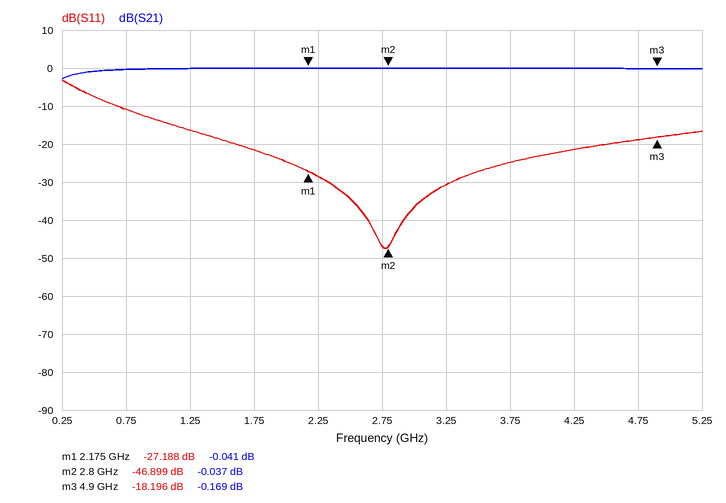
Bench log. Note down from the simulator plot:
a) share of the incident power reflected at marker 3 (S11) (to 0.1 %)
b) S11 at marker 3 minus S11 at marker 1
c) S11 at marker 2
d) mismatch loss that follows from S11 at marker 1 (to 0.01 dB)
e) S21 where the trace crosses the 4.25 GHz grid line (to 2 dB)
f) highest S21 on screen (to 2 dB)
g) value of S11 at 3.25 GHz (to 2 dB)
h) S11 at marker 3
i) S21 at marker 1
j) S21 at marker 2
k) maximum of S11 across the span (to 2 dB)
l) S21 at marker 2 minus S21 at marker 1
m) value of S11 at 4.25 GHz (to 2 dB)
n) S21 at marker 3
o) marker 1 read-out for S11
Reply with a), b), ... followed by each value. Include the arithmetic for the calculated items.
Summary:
a) 10^(-18.196/10) ≈ 1.5 %
b) -18.196 − (-27.188) = 8.992 dB
c) -46.899 dB
d) −10 log10(1 − 10^(-27.188/10)) ≈ 0.01 dB
e) 0 dB
f) 0 dB
g) -30 dB
h) -18.196 dB
i) -0.041 dB
j) -0.037 dB
k) -4 dB
l) -0.037 − (-0.041) = 0.004 dB
m) -22 dB
n) -0.169 dB
o) -27.188 dB
